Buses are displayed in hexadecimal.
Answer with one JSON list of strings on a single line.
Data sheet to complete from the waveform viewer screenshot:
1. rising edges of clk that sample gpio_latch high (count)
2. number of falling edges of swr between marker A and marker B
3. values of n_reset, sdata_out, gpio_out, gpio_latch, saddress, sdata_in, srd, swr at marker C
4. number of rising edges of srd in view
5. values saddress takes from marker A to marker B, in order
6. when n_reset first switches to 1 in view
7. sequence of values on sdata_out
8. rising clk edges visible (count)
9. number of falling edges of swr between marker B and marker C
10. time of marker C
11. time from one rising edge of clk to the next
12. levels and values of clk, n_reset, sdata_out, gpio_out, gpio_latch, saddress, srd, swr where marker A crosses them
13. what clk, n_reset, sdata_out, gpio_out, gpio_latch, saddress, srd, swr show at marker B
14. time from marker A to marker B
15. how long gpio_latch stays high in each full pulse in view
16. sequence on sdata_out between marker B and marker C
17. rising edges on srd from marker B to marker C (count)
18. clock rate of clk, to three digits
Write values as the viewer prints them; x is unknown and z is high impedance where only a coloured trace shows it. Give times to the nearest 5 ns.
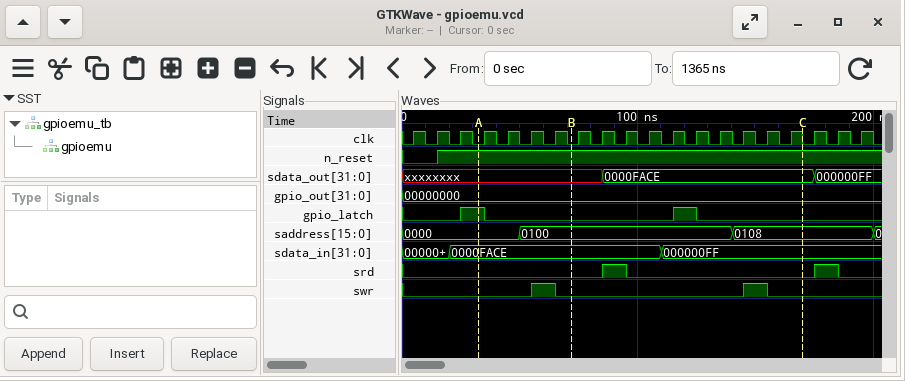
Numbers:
["2", "1", "n_reset=1, sdata_out=0000FACE, gpio_out=00000000, gpio_latch=0, saddress=0108, sdata_in=000000FF, srd=0, swr=0", "2", "0000, 0100", "15 ns", "xxxxxxxx, 0000FACE, 000000FF", "20", "1", "170 ns", "10 ns", "clk=0, n_reset=1, sdata_out=xxxxxxxx, gpio_out=00000000, gpio_latch=1, saddress=0000, srd=0, swr=0", "clk=0, n_reset=1, sdata_out=xxxxxxxx, gpio_out=00000000, gpio_latch=0, saddress=0100, srd=0, swr=0", "40 ns", "10 ns, 10 ns", "xxxxxxxx, 0000FACE", "1", "100 MHz"]
